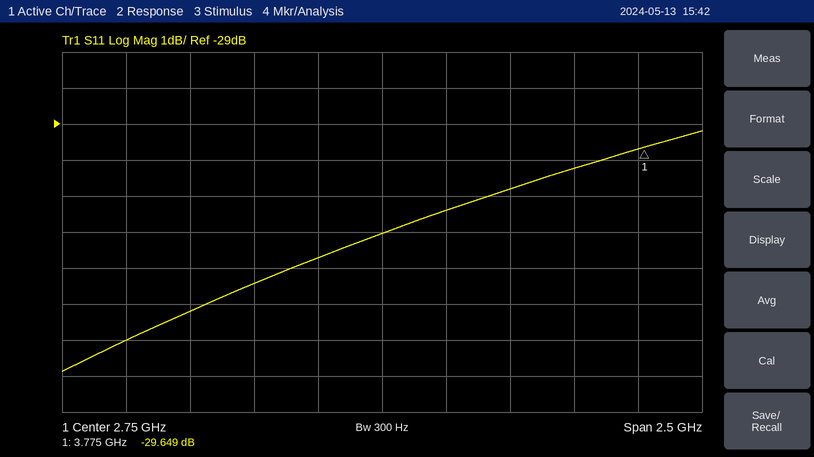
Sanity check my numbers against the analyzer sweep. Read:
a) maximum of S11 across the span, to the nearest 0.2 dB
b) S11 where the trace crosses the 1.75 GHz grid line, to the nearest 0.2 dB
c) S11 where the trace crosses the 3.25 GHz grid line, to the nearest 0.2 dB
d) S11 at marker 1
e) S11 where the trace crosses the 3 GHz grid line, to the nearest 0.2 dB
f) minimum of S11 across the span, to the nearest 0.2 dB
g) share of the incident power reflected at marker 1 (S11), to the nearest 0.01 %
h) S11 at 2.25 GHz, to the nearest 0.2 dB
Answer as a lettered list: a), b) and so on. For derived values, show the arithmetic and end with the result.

a) -29.2 dB
b) -35.0 dB
c) -30.8 dB
d) -29.649 dB
e) -31.4 dB
f) -35.8 dB
g) 10^(-29.649/10) ≈ 0.11 %
h) -33.4 dB
